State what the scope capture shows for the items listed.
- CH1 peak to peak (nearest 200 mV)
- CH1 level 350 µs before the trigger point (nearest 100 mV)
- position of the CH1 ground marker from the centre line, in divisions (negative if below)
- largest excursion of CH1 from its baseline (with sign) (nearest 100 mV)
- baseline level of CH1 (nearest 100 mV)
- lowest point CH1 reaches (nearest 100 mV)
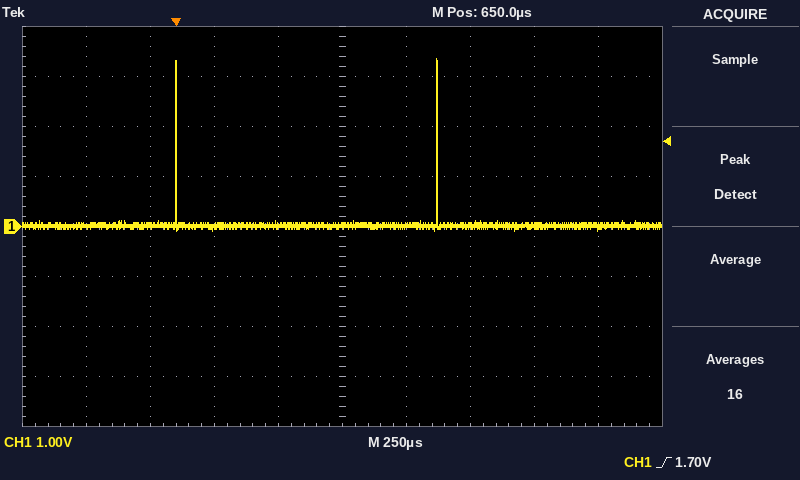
3.4 V
0.0 V
0.0 div
+3.3 V
0.0 V
-100 mV
